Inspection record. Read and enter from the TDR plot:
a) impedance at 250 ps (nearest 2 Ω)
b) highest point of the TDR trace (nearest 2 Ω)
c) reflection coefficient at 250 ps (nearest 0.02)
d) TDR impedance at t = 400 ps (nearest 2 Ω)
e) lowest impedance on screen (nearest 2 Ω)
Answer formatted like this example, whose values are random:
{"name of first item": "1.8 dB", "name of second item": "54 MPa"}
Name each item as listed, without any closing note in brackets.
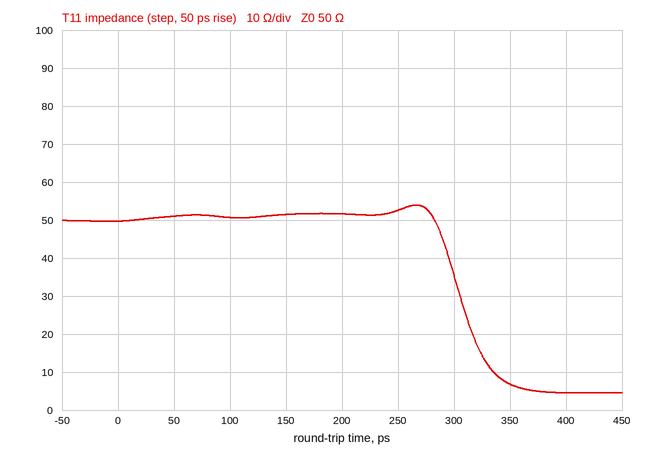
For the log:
{"impedance at 250 ps": "52 Ω", "highest point of the TDR trace": "54 Ω", "reflection coefficient at 250 ps": "+0.02", "TDR impedance at t = 400 ps": "4 Ω", "lowest impedance on screen": "4 Ω"}
